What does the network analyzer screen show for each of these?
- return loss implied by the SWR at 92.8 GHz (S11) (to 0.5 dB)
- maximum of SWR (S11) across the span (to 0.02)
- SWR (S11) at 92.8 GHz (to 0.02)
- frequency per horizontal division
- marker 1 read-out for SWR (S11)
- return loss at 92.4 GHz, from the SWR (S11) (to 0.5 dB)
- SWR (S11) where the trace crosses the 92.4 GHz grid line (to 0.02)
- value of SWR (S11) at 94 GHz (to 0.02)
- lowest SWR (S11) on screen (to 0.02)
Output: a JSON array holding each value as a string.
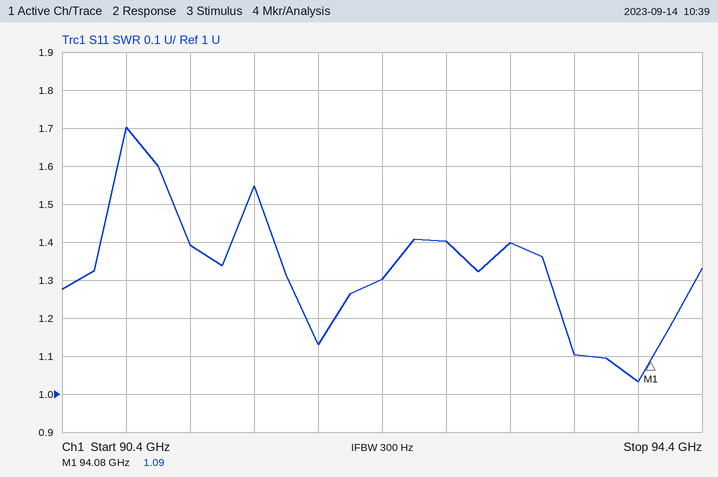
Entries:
["15.5 dB", "1.70", "1.40", "400 MHz", "1.09", "17.5 dB", "1.30", "1.04", "1.04"]
